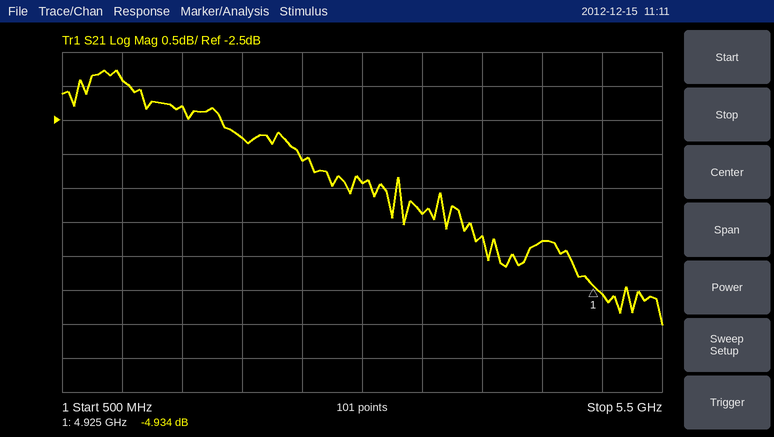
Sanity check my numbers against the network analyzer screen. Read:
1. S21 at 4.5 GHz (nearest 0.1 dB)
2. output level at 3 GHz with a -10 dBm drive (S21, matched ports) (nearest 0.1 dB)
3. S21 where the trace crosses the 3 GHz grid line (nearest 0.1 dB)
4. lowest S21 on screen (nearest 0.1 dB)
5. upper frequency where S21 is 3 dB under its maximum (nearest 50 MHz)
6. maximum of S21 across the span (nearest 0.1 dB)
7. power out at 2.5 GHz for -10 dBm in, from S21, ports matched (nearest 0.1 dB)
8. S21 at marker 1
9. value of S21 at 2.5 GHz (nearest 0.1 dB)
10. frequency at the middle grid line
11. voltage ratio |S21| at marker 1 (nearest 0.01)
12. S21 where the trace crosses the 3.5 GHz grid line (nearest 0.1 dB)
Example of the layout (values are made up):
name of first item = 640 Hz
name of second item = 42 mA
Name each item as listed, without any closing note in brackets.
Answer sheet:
S21 at 4.5 GHz = -4.3 dB
output level at 3 GHz with a -10 dBm drive (S21, matched ports) = -13.4 dBm
S21 where the trace crosses the 3 GHz grid line = -3.4 dB
lowest S21 on screen = -5.5 dB
upper frequency where S21 is 3 dB under its maximum = 4.80 GHz
maximum of S21 across the span = -1.8 dB
power out at 2.5 GHz for -10 dBm in, from S21, ports matched = -13.1 dBm
S21 at marker 1 = -4.934 dB
value of S21 at 2.5 GHz = -3.1 dB
frequency at the middle grid line = 3 GHz
voltage ratio |S21| at marker 1 = 0.57
S21 where the trace crosses the 3.5 GHz grid line = -3.9 dB
